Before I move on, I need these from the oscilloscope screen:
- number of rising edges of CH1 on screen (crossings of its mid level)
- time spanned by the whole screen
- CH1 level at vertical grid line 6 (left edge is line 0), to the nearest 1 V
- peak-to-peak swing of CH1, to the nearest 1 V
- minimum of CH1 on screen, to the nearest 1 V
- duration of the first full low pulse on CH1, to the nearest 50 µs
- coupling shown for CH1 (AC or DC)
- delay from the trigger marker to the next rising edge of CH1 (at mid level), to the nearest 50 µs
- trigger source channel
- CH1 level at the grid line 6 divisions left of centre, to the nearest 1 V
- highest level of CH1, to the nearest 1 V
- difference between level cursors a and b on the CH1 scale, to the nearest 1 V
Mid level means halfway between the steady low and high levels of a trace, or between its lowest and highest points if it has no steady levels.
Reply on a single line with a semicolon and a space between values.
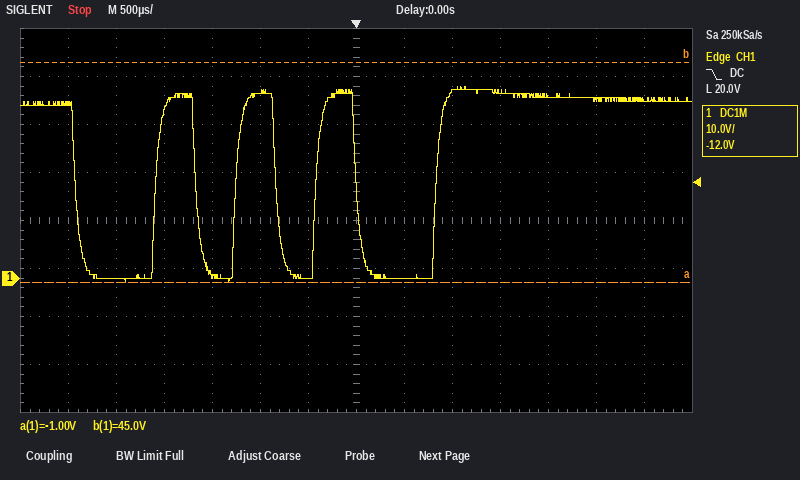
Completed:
4; 7 ms; 0 V; 41 V; -1 V; 850 µs; DC; 850 µs; CH1; 36 V; 40 V; 46 V
